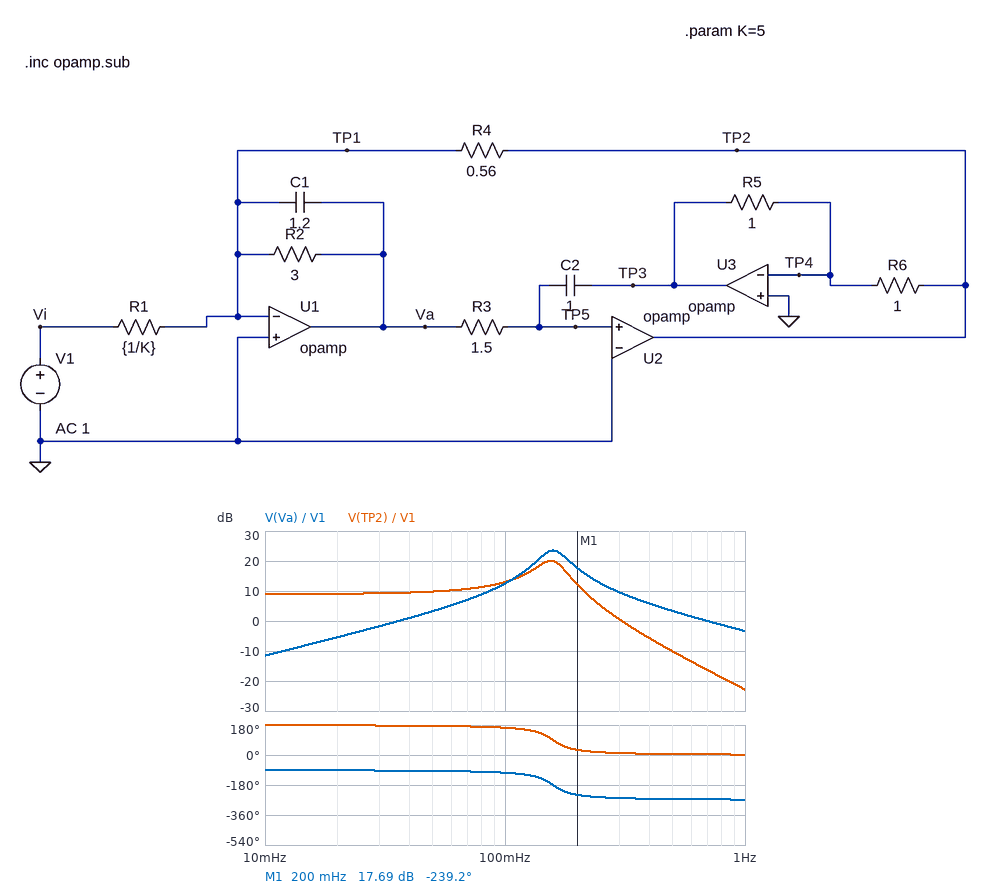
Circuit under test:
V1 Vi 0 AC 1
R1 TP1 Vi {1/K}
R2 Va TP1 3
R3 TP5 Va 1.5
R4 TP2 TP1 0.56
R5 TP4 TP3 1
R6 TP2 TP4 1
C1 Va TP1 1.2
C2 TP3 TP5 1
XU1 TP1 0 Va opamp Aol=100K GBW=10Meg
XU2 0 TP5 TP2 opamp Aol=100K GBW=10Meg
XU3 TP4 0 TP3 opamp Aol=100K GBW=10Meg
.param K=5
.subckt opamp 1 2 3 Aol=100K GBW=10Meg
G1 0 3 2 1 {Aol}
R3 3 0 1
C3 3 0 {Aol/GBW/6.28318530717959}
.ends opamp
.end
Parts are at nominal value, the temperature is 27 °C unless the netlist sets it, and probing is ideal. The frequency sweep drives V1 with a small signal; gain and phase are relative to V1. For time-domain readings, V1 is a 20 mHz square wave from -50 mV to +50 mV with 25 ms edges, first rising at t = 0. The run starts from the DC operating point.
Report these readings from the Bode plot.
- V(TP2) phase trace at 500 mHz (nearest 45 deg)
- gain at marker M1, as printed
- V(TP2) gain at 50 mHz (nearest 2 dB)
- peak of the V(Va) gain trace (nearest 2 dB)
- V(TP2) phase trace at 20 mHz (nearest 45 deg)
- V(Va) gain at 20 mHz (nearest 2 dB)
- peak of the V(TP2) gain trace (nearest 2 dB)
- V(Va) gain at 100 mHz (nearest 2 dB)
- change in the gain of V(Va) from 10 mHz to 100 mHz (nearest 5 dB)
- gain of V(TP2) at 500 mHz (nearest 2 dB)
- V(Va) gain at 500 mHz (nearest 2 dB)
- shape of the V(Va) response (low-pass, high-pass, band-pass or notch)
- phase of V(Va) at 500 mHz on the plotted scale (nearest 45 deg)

0 deg
17.69 dB
10 dB
24 dB
180 deg
-6 dB
20 dB
12 dB
25 dB
-10 dB
4 dB
band-pass
-270 deg
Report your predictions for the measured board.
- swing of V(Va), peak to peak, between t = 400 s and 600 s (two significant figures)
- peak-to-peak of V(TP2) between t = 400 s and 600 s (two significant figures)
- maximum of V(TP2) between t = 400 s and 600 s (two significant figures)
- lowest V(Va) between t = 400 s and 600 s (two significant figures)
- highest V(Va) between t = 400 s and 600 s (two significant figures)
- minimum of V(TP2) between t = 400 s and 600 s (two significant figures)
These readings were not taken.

670 mV
630 mV
320 mV
-330 mV
330 mV
-320 mV
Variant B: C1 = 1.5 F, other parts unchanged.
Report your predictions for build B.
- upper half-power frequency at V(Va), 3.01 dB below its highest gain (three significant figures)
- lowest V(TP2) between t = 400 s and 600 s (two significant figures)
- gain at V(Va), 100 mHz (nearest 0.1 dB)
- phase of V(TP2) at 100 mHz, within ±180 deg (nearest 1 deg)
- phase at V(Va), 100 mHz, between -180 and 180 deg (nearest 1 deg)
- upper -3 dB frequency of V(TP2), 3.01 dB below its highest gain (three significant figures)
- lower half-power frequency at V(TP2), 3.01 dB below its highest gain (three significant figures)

161 mHz
-340 mV
13.9 dB
161 deg
-109 deg
156 mHz
120 mHz
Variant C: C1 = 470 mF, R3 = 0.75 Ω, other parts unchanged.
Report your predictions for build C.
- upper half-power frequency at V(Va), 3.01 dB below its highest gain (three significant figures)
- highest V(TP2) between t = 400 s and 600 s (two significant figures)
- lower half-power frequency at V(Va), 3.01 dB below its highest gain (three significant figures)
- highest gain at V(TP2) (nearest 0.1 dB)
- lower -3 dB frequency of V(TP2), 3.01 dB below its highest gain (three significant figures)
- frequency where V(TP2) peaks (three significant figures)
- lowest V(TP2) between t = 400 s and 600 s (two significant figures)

419 mHz
310 mV
306 mHz
19.1 dB
286 mHz
349 mHz
-310 mV
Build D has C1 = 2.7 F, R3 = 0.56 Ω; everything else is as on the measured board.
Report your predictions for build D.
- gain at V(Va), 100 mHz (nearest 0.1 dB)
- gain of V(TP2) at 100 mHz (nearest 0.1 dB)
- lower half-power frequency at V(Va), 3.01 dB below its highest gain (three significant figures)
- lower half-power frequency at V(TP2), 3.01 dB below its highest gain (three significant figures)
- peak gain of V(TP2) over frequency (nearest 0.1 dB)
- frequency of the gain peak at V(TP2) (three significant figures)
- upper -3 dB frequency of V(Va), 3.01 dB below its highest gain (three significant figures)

3.4 dB
12.4 dB
163 mHz
162 mHz
27.8 dB
172 mHz
183 mHz
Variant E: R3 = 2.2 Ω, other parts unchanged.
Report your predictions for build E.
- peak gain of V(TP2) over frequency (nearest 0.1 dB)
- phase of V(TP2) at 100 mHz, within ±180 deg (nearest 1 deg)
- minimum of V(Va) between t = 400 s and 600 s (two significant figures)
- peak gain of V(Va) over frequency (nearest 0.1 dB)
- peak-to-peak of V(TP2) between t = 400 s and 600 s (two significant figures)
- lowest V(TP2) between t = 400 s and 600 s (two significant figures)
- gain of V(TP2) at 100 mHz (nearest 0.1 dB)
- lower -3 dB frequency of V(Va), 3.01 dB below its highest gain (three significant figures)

18.5 dB
148 deg
-390 mV
23.5 dB
600 mV
-300 mV
15.1 dB
111 mHz
